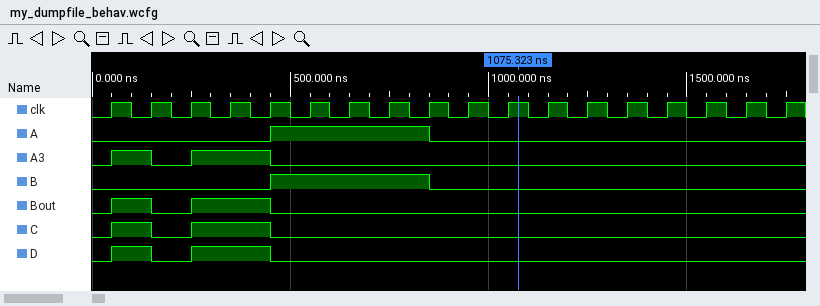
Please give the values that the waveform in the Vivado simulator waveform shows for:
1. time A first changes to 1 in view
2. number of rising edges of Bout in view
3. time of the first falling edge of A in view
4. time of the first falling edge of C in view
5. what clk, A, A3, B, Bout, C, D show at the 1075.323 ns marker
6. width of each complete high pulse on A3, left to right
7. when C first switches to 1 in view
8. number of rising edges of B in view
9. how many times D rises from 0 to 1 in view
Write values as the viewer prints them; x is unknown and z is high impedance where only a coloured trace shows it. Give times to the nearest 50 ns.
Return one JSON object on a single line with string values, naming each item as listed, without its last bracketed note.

{"time A first changes to 1 in view": "450 ns", "number of rising edges of Bout in view": "2", "time of the first falling edge of A in view": "850 ns", "time of the first falling edge of C in view": "150 ns", "what clk, A, A3, B, Bout, C, D show at the 1075.323 ns marker": "clk=1, A=0, A3=0, B=0, Bout=0, C=0, D=0", "width of each complete high pulse on A3, left to right": "100 ns, 200 ns", "when C first switches to 1 in view": "50 ns", "number of rising edges of B in view": "1", "how many times D rises from 0 to 1 in view": "2"}
